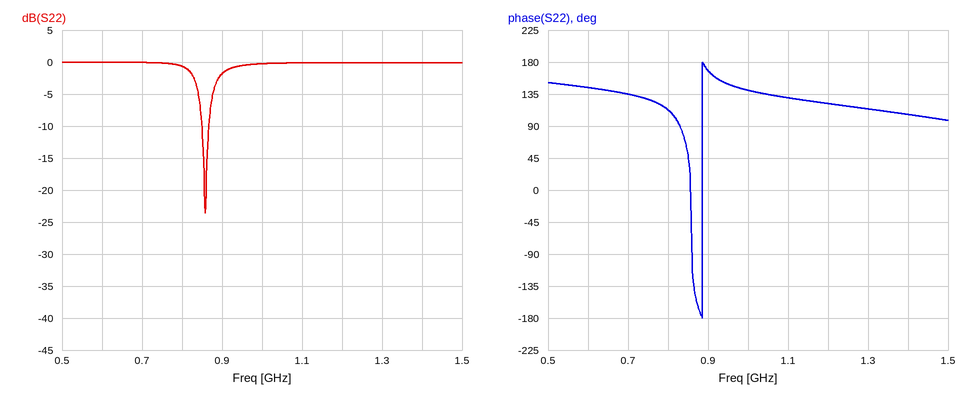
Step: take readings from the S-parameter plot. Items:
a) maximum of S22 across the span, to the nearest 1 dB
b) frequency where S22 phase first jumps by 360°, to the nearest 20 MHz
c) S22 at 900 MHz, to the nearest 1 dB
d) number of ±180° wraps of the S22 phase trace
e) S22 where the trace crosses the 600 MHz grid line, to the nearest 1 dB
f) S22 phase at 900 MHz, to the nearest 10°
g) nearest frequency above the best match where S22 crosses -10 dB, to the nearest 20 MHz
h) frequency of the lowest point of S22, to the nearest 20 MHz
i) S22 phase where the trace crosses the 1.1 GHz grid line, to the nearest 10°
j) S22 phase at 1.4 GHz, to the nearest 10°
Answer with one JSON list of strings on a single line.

["0 dB", "880 MHz", "-2 dB", "1", "0 dB", "170°", "860 MHz", "860 MHz", "130°", "110°"]
